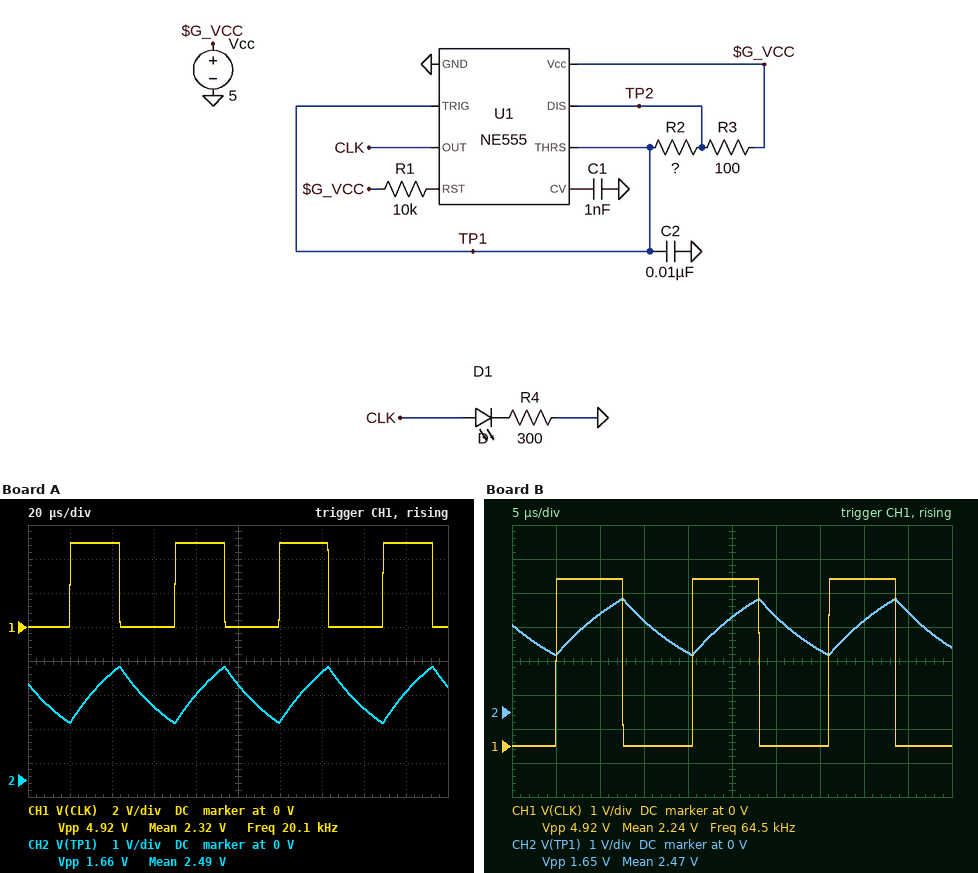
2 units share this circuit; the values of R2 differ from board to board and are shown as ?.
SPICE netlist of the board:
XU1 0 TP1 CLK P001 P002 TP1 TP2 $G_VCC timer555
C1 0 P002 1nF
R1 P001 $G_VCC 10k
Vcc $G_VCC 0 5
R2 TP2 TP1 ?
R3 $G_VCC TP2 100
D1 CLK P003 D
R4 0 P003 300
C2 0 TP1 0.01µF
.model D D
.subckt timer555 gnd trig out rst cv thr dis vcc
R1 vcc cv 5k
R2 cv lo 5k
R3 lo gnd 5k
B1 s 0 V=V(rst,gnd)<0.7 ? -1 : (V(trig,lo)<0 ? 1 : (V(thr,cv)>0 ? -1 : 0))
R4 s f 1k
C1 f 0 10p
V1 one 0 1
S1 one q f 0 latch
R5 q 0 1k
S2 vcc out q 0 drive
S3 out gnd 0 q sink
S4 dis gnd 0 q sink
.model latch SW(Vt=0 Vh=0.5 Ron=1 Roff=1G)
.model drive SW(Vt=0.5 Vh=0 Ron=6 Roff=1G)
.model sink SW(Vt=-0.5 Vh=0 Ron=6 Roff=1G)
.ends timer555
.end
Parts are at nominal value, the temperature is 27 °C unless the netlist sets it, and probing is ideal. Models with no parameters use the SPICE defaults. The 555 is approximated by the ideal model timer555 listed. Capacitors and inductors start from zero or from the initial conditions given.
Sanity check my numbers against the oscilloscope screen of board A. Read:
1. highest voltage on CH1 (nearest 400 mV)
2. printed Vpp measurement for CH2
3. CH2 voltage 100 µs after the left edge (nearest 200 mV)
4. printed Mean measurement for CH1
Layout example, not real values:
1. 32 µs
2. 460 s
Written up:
1. 4.8 V
2. 1.66 V
3. 2.8 V
4. 2.32 V
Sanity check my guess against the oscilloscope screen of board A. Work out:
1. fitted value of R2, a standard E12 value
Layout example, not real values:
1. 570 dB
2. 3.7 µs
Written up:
1. 3.3 kΩ
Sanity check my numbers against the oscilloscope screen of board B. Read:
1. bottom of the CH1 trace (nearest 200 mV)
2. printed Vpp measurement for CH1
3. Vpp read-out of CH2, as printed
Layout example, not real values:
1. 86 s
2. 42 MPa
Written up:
1. 0 V
2. 4.92 V
3. 1.65 V
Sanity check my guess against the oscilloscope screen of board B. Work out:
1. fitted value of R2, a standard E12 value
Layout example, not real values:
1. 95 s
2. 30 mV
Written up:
1. 1 kΩ
